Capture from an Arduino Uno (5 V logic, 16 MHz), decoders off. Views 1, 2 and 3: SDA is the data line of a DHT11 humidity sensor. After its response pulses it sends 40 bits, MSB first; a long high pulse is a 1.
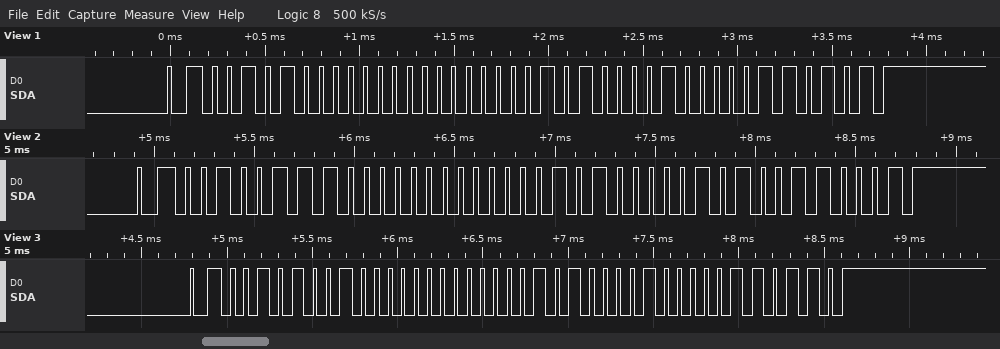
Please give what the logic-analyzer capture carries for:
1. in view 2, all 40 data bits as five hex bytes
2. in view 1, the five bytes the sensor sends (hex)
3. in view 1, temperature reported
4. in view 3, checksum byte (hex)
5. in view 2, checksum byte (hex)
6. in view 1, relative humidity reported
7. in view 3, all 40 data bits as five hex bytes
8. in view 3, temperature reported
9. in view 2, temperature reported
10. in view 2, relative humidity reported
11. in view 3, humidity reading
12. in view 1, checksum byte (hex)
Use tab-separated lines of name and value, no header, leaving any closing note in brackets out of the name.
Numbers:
in view 2, all 40 data bits as five hex bytes	27 00 05 05 31
in view 1, the five bytes the sensor sends	28 00 05 08 35
in view 1, temperature reported	5.8 °C
in view 3, checksum byte	0x36
in view 2, checksum byte	0x31
in view 1, relative humidity reported	40 %
in view 3, all 40 data bits as five hex bytes	29 00 05 08 36
in view 3, temperature reported	5.8 °C
in view 2, temperature reported	5.5 °C
in view 2, relative humidity reported	39 %
in view 3, humidity reading	41 %
in view 1, checksum byte	0x35
